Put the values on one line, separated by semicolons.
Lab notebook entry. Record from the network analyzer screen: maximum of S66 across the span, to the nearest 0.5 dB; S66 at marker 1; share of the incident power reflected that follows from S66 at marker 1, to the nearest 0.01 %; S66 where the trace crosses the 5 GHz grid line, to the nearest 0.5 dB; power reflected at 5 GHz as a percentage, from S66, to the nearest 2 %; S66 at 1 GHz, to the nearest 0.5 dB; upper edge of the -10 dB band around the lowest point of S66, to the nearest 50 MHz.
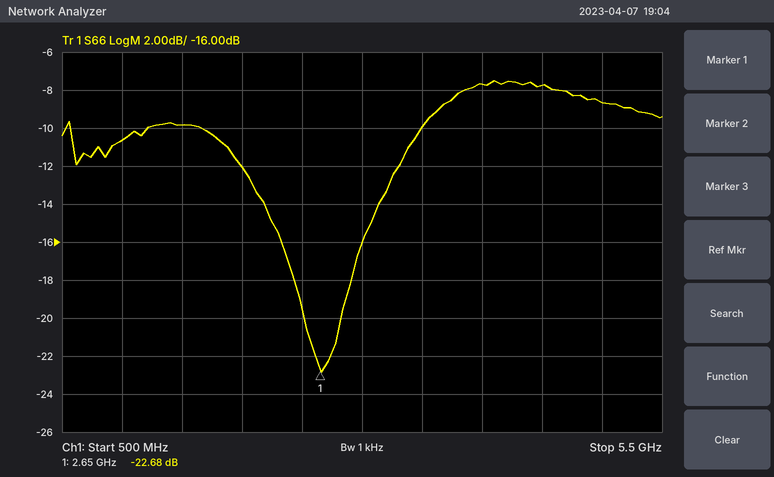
-7.5 dB; -22.68 dB; 0.54 %; -8.5 dB; 14 %; -10.5 dB; 3.50 GHz
